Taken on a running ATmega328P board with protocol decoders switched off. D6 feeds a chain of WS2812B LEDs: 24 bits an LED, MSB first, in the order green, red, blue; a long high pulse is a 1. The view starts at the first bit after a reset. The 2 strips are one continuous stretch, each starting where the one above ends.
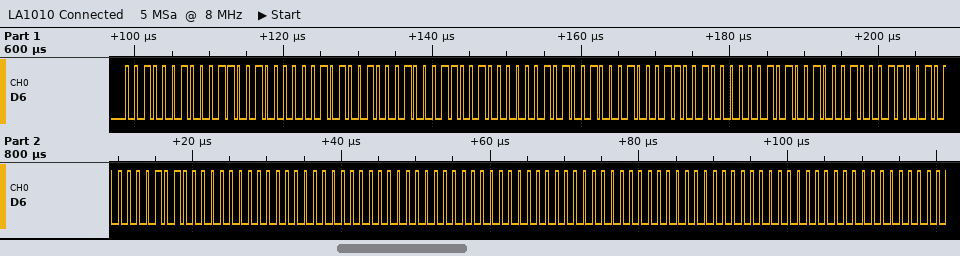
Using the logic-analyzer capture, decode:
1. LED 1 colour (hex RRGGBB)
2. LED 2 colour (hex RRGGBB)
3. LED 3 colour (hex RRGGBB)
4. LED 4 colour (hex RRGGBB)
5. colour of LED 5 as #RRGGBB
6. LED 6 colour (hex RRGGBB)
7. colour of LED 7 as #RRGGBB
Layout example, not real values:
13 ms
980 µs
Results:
#322205
#322205
#322205
#322205
#000000
#000000
#000000
